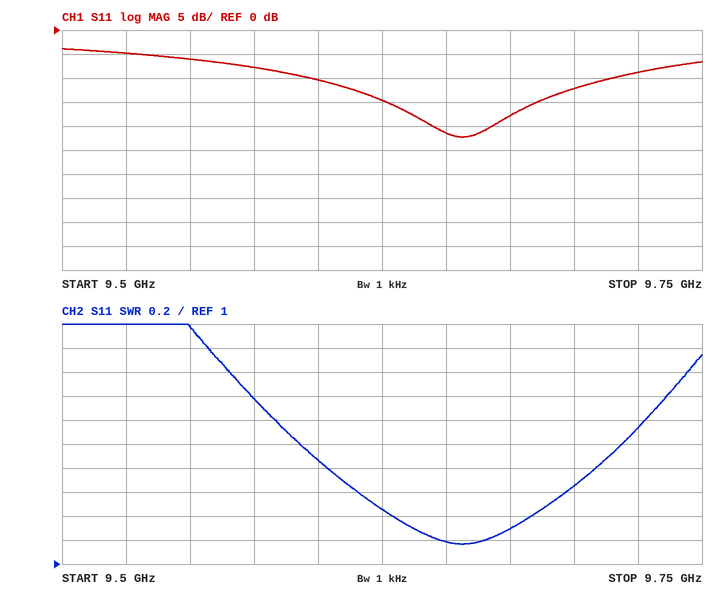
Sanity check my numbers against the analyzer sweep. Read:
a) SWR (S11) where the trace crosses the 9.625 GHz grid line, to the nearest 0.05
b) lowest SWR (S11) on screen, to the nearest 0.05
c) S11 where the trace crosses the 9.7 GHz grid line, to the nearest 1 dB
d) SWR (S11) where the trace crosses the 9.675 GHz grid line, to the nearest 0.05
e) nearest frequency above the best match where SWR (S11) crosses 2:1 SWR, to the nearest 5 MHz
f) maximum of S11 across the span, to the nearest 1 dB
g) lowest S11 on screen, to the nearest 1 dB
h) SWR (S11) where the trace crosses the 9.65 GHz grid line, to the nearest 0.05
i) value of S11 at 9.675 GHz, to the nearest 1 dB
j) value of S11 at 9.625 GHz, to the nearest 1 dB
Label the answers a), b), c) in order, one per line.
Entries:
a) 1.45
b) 1.15
c) -12 dB
d) 1.30
e) 9.720 GHz
f) -4 dB
g) -22 dB
h) 1.20
i) -18 dB
j) -15 dB
